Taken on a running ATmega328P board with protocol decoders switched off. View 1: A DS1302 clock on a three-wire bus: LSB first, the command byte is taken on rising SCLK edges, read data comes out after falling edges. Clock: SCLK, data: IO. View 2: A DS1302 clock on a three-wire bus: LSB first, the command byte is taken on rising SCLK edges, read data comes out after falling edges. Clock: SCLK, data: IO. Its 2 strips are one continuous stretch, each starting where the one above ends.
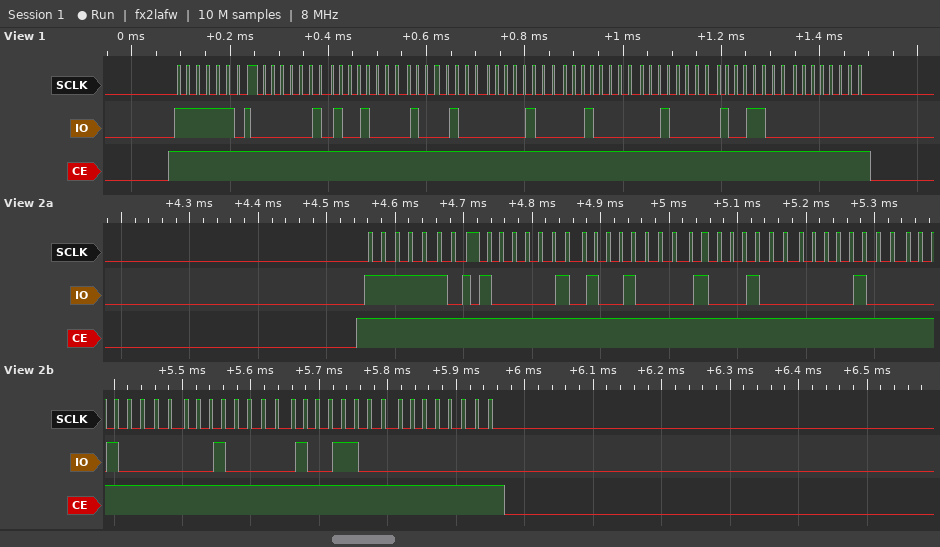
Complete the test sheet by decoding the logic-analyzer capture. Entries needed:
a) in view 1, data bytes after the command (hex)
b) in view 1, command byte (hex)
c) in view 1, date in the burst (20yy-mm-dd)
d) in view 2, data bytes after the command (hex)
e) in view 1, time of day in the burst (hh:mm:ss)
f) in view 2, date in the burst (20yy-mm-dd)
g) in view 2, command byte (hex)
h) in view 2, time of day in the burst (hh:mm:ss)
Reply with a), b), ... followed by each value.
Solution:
a) 40 09 11 10 04 04 19 00
b) 0xBF
c) 2019-04-10
d) 41 09 11 10 04 04 19 00
e) 11:09:40
f) 2019-04-10
g) 0xBF
h) 11:09:41
